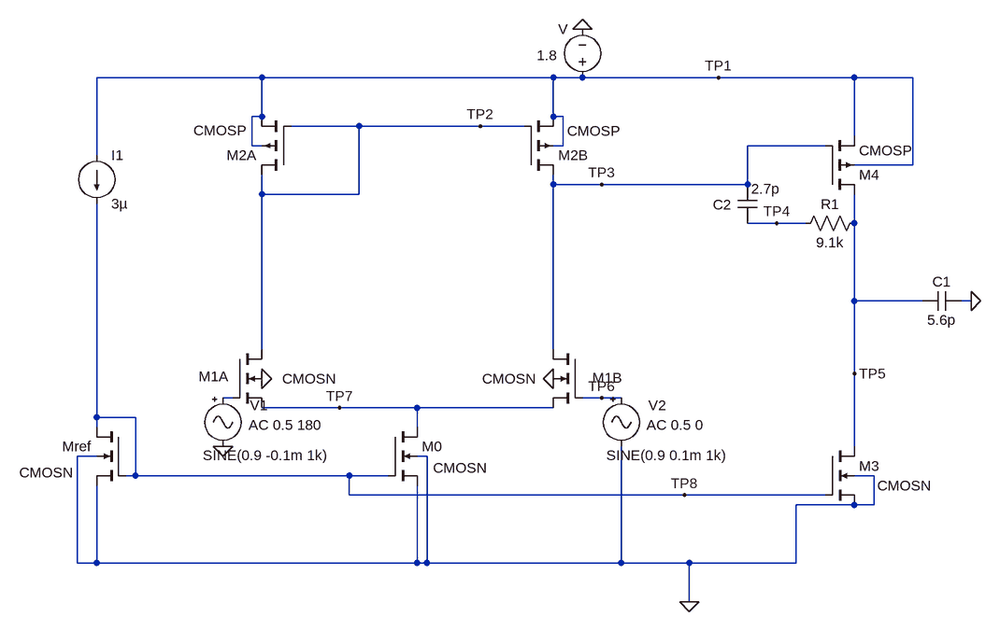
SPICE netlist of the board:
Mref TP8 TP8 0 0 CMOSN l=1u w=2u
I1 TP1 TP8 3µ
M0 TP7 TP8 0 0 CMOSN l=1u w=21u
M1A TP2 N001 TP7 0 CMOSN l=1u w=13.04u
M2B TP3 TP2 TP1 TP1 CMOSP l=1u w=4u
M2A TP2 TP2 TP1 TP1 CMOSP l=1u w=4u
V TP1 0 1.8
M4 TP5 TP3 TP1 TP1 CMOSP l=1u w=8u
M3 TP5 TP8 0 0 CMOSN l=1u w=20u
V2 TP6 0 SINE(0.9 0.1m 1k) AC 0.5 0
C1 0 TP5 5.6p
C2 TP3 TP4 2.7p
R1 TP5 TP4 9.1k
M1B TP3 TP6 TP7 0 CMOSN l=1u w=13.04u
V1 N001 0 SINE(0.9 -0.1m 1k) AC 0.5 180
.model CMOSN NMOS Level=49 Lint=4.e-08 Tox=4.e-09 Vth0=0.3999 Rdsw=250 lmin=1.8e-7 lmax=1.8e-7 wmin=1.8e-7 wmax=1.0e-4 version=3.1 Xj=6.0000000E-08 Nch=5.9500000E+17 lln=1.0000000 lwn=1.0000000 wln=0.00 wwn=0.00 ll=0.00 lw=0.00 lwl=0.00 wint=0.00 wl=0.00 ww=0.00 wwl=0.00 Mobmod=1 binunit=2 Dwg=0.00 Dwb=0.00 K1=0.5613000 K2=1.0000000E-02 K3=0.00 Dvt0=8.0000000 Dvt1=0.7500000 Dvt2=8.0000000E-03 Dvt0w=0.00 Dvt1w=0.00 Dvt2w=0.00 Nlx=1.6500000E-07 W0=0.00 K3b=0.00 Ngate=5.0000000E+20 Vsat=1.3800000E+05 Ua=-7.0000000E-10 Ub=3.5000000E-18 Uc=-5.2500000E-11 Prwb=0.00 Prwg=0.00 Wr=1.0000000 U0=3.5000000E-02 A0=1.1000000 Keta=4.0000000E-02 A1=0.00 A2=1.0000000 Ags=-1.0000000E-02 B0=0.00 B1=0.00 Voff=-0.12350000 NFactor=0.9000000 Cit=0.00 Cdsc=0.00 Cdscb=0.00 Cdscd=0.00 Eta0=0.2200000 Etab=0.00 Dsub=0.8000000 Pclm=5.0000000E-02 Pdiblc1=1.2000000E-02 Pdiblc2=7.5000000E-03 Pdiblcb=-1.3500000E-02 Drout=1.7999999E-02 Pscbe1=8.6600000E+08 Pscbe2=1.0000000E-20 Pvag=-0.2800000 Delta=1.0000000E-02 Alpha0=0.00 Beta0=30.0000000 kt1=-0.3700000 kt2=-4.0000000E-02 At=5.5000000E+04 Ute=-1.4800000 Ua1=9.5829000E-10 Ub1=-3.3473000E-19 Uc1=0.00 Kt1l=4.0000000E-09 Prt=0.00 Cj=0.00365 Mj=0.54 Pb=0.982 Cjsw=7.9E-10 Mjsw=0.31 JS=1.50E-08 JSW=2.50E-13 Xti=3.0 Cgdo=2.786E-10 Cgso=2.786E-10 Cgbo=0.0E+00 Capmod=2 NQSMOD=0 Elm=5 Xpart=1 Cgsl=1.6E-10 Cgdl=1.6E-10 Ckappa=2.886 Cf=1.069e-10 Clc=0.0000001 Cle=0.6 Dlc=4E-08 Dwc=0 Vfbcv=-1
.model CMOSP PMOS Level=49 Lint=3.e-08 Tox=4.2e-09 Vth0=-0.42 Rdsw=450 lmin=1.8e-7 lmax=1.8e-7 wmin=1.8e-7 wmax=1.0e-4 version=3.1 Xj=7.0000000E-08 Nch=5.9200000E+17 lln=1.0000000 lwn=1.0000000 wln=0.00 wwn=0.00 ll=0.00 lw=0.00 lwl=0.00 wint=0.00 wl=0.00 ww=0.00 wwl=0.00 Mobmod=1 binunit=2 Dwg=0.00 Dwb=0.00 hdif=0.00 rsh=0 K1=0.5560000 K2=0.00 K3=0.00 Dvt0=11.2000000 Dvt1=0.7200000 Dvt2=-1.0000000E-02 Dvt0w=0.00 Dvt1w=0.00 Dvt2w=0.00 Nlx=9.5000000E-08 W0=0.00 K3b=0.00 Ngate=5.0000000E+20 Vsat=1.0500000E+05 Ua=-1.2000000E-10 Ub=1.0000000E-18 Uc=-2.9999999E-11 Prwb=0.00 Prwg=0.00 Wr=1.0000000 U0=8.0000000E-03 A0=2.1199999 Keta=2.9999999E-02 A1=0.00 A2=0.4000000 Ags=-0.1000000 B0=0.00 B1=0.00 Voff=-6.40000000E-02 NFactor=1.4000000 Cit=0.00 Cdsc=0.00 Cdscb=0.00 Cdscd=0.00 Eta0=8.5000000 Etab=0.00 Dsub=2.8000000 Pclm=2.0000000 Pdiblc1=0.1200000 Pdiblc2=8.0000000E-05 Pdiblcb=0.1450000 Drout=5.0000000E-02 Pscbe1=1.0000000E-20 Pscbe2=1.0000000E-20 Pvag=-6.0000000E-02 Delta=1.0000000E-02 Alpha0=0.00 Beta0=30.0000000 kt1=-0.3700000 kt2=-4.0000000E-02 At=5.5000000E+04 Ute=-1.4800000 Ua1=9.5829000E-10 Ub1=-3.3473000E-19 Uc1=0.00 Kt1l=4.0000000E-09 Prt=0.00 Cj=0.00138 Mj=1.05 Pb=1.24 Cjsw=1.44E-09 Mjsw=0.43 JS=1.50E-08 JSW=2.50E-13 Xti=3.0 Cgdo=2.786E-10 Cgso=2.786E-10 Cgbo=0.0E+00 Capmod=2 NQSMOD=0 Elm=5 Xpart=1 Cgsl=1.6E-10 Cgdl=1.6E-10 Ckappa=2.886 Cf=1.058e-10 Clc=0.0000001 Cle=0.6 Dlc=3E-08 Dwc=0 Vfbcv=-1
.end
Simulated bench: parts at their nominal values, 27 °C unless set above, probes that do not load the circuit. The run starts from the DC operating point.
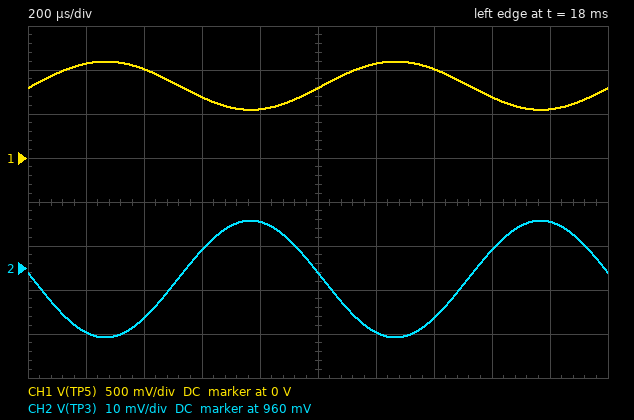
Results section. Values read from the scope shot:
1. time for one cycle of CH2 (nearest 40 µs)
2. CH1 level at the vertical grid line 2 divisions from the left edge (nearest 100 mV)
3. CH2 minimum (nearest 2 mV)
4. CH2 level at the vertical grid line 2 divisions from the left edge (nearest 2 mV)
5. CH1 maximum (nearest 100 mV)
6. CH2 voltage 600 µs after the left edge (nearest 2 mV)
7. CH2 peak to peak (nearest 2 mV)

1.00 ms
1.0 V
944 mV
948 mV
1.1 V
964 mV
26 mV
